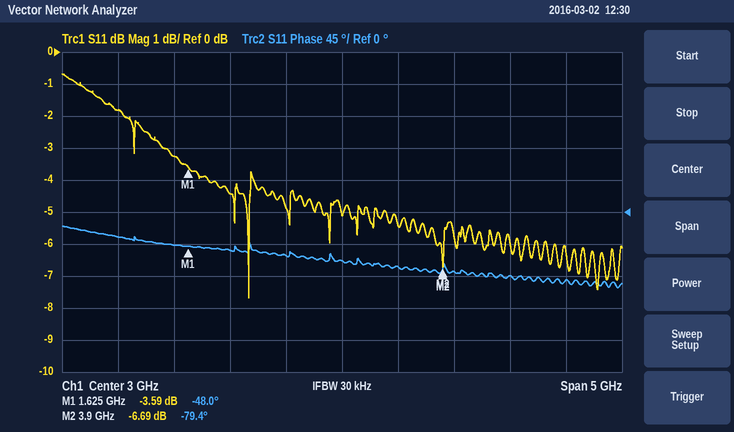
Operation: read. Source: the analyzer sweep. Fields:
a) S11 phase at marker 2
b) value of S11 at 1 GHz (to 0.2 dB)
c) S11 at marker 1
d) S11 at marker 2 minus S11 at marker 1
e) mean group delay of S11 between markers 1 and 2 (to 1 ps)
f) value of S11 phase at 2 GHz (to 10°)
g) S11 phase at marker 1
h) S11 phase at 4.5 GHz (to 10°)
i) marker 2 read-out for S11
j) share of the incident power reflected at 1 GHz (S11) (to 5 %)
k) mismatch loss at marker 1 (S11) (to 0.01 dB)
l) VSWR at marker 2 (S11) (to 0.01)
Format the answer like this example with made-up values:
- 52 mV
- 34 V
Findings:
- -79.4°
- -1.8 dB
- -3.59 dB
- -3.10 dB
- 38 ps
- -50°
- -48.0°
- -90°
- -6.69 dB
- 65 %
- 2.50 dB
- 2.72
